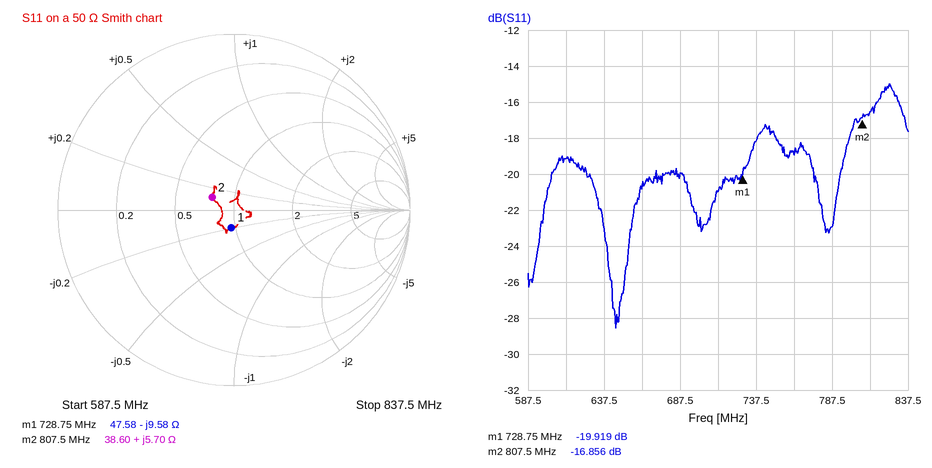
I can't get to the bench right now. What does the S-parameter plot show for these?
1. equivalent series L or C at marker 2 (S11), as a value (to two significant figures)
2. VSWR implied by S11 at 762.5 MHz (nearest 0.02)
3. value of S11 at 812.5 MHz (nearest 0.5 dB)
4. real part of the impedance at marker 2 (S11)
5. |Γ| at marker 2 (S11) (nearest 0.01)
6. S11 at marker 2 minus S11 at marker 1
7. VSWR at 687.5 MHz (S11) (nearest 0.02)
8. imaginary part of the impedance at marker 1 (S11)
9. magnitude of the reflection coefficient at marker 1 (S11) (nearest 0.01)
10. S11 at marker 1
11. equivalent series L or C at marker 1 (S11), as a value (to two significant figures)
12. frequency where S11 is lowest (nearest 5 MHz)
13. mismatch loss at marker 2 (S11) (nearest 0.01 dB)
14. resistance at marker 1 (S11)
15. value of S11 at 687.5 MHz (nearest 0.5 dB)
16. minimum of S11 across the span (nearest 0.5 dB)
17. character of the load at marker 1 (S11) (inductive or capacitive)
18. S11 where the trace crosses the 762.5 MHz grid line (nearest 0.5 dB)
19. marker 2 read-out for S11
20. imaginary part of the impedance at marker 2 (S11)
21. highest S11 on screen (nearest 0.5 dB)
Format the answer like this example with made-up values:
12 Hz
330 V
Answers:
1.1 nH
1.26
-16.5 dB
38.60 Ω
0.14
3.063 dB
1.22
-9.58 Ω
0.10
-19.919 dB
23 pF
645 MHz
0.09 dB
47.58 Ω
-20.0 dB
-28.5 dB
capacitive
-19.0 dB
-16.856 dB
+5.70 Ω
-15.0 dB
